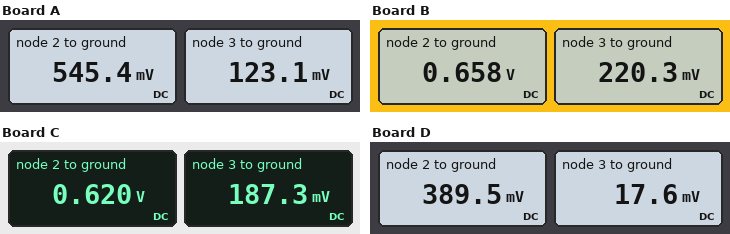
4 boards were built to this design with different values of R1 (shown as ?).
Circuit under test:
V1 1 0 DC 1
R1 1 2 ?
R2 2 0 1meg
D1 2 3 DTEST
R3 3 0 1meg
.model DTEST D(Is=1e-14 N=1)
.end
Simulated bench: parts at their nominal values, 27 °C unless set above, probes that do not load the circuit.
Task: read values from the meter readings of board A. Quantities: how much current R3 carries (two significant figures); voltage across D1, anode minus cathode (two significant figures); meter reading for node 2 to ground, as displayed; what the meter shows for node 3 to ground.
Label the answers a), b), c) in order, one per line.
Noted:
a) 120 nA
b) 420 mV
c) 545.4 mV
d) 123.1 mV
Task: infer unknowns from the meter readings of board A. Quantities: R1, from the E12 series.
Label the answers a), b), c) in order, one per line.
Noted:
a) 680 kΩ
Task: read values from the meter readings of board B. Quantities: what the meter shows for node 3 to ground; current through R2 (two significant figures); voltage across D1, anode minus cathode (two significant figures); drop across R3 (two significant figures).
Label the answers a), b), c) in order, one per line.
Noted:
a) 220.3 mV
b) 660 nA
c) 440 mV
d) 220 mV
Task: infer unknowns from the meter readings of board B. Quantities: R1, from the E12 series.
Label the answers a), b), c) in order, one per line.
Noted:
a) 390 kΩ
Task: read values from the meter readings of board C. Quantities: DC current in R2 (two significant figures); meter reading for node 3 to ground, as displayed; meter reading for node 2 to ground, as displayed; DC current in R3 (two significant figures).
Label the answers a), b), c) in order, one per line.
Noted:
a) 620 nA
b) 187.3 mV
c) 0.620 V
d) 190 nA
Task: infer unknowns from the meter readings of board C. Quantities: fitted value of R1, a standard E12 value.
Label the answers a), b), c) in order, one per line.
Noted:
a) 470 kΩ
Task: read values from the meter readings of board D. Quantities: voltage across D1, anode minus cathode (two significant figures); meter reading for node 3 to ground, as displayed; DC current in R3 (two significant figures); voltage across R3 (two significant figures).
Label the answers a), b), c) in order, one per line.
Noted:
a) 370 mV
b) 17.6 mV
c) 18 nA
d) 18 mV
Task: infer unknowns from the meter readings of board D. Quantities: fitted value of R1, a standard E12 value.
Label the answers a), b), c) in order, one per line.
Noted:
a) 1.5 MΩ
